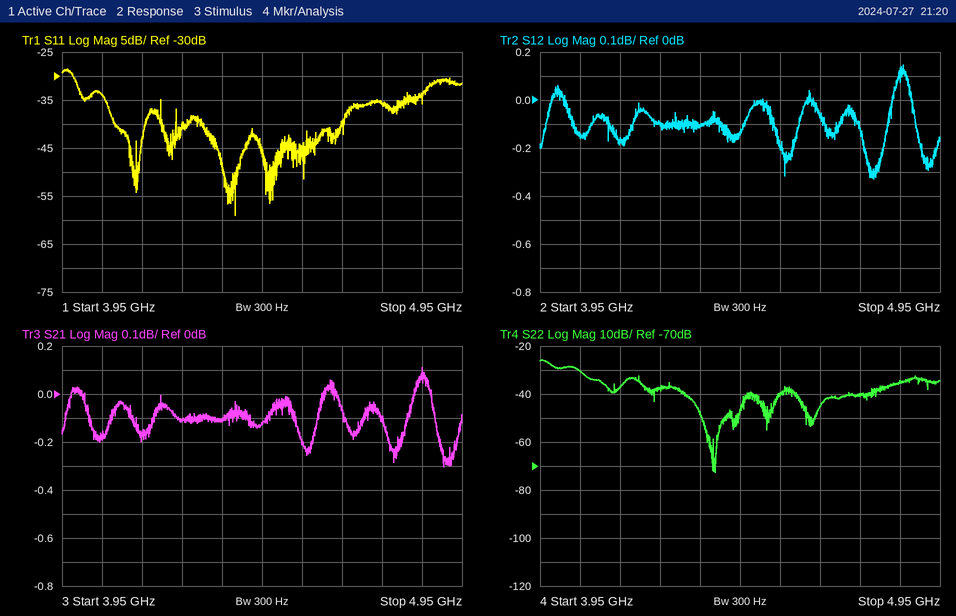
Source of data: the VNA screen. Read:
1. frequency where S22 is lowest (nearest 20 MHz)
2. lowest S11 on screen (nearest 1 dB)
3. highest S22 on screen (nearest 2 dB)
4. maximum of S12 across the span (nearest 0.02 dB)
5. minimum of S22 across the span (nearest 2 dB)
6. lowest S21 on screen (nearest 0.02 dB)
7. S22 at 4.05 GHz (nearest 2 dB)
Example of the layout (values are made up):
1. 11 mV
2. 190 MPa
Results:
1. 4.38 GHz
2. -59 dB
3. -26 dB
4. 0.14 dB
5. -72 dB
6. -0.30 dB
7. -30 dB
